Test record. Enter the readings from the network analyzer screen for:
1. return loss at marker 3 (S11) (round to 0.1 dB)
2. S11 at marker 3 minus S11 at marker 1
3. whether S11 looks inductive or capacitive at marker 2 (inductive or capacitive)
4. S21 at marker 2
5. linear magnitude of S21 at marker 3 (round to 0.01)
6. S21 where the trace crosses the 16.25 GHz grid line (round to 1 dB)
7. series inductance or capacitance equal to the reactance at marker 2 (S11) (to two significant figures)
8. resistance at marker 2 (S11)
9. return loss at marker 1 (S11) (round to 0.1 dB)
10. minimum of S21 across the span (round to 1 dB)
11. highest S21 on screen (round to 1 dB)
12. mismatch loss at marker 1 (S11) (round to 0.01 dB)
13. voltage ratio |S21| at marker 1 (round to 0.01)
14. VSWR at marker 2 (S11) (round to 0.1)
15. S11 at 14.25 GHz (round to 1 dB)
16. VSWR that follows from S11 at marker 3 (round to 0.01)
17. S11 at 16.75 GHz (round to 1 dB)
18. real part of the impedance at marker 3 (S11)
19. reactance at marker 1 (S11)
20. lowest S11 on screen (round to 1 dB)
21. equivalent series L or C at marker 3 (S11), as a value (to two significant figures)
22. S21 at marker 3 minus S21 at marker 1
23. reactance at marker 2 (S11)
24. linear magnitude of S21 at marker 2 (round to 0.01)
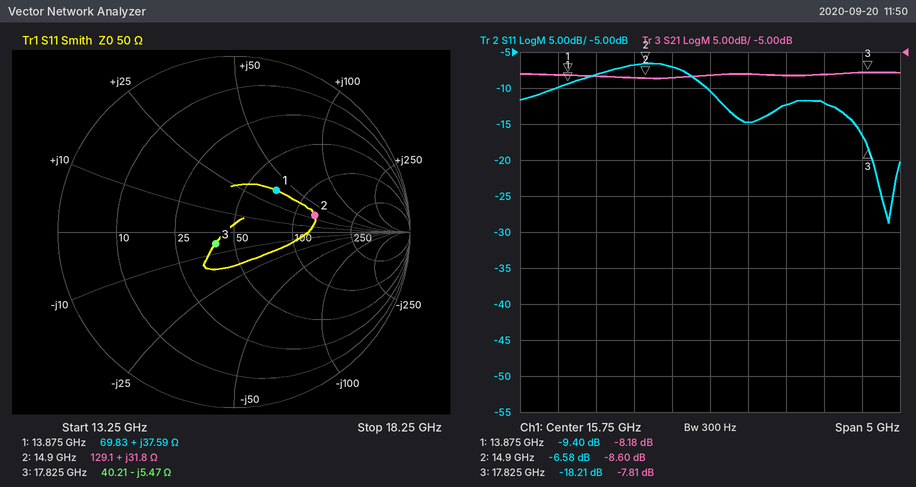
18.1 dB
-8.81 dB
inductive
-8.60 dB
0.41
-8 dB
340 pH
129.1 Ω
9.4 dB
-9 dB
-8 dB
0.53 dB
0.39
2.8
-8 dB
1.28
-12 dB
40.21 Ω
+37.59 Ω
-29 dB
1.6 pF
0.37 dB
+31.8 Ω
0.37
